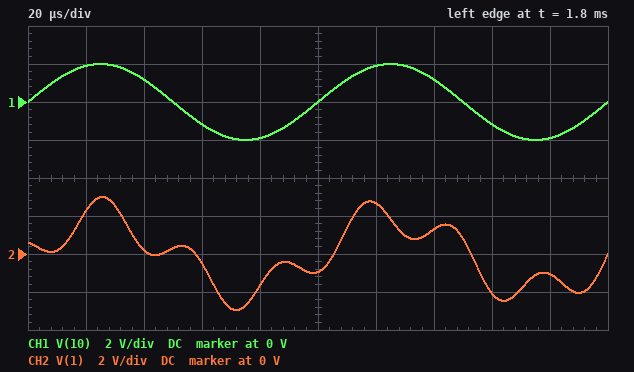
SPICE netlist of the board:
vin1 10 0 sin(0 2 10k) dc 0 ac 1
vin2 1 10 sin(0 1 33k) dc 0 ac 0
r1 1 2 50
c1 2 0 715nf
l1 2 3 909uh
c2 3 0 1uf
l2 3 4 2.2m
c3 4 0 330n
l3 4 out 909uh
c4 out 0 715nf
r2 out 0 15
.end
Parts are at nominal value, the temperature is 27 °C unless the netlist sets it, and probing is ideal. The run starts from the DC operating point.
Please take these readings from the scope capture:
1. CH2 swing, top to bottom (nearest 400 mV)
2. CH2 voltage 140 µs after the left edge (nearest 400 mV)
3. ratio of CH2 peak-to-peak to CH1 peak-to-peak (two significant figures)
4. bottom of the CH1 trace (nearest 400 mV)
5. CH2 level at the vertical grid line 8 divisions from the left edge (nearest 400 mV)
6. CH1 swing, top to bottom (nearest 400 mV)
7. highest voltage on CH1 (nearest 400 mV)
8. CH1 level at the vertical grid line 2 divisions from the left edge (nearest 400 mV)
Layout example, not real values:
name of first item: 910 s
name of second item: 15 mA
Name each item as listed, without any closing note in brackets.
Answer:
CH2 swing, top to bottom: 6.0 V
CH2 voltage 140 µs after the left edge: 1.2 V
ratio of CH2 peak-to-peak to CH1 peak-to-peak: 1.5
bottom of the CH1 trace: -2.0 V
CH2 level at the vertical grid line 8 divisions from the left edge: -2.0 V
CH1 swing, top to bottom: 4.0 V
highest voltage on CH1: 2.0 V
CH1 level at the vertical grid line 2 divisions from the left edge: 1.2 V
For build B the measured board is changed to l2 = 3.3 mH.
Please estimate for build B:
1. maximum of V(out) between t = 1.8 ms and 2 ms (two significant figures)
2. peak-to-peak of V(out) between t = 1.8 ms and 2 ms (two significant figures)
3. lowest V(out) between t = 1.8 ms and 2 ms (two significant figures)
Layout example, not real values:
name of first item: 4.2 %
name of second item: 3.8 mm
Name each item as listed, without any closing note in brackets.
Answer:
maximum of V(out) between t = 1.8 ms and 2 ms: 130 mV
peak-to-peak of V(out) between t = 1.8 ms and 2 ms: 260 mV
lowest V(out) between t = 1.8 ms and 2 ms: -130 mV
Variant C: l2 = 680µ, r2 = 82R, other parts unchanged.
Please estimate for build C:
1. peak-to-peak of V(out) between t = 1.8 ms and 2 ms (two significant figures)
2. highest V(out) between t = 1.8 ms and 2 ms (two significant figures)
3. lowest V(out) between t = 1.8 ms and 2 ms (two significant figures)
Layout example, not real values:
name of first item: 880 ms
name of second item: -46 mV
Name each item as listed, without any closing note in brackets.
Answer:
peak-to-peak of V(out) between t = 1.8 ms and 2 ms: 560 mV
highest V(out) between t = 1.8 ms and 2 ms: 280 mV
lowest V(out) between t = 1.8 ms and 2 ms: -280 mV
